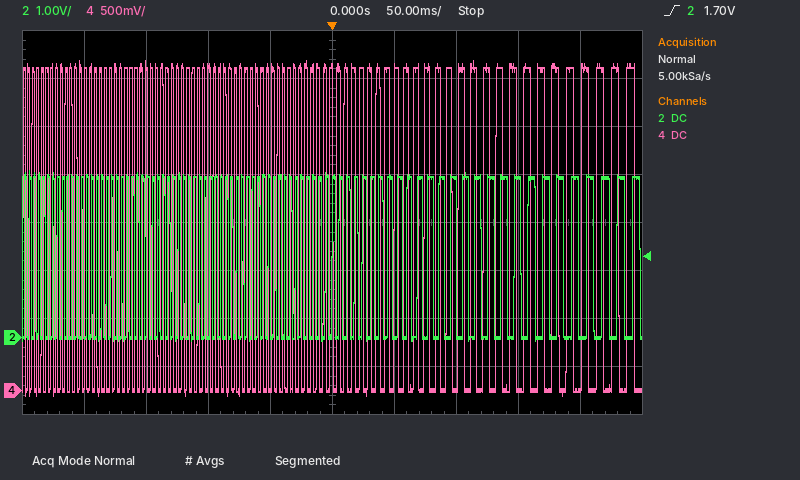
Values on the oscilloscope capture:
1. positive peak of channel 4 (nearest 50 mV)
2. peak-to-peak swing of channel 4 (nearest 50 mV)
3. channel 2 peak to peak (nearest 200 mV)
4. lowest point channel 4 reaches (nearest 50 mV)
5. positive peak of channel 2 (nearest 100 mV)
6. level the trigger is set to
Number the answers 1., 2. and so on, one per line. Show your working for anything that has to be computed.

1. 3.45 V
2. 3.45 V − (-50 mV) = 3.50 V
3. 3.6 V
4. -50 mV
5. 3.5 V
6. 1.70 V
